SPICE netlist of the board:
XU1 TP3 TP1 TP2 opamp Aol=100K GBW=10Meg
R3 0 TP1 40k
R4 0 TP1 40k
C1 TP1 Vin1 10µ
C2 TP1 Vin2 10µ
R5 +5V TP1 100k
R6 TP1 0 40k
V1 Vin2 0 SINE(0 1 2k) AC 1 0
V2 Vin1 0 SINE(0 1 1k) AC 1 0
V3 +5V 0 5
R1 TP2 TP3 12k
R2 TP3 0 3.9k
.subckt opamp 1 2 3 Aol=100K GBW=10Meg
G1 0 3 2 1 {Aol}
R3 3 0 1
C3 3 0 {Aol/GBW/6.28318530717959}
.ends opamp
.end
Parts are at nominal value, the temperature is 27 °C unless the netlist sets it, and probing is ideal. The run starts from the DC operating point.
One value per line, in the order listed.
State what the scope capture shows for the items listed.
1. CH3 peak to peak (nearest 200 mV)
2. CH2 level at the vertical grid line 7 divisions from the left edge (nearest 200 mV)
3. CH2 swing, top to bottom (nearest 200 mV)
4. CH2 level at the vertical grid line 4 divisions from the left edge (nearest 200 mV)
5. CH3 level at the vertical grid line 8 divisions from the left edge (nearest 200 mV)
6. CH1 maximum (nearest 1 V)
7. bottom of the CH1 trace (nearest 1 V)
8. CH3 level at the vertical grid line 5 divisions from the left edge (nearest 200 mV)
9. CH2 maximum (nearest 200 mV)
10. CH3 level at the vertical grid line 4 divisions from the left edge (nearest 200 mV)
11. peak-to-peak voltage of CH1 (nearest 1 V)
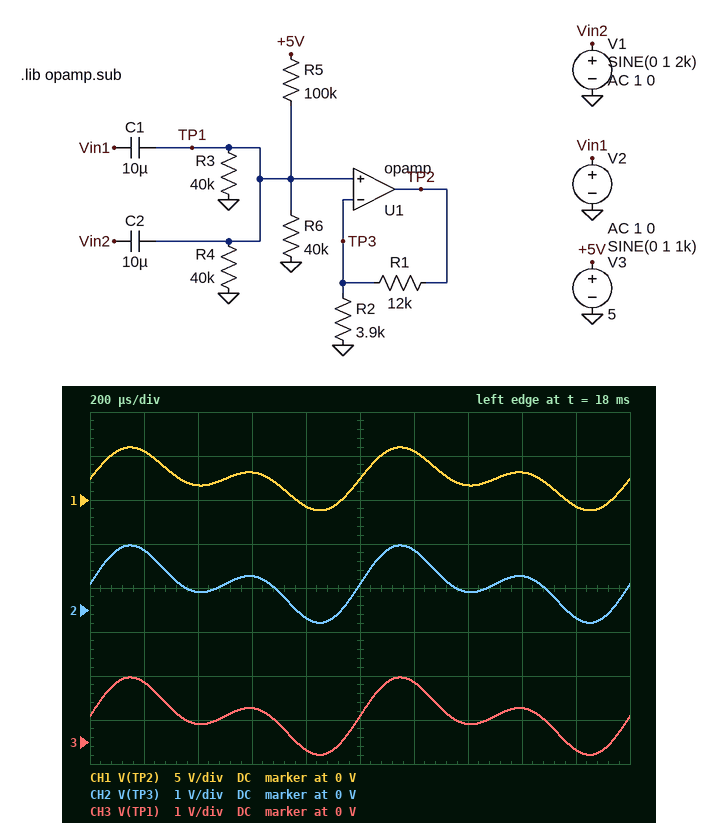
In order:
1.8 V
400 mV
1.8 V
-200 mV
800 mV
6 V
-1 V
600 mV
1.4 V
-200 mV
7 V
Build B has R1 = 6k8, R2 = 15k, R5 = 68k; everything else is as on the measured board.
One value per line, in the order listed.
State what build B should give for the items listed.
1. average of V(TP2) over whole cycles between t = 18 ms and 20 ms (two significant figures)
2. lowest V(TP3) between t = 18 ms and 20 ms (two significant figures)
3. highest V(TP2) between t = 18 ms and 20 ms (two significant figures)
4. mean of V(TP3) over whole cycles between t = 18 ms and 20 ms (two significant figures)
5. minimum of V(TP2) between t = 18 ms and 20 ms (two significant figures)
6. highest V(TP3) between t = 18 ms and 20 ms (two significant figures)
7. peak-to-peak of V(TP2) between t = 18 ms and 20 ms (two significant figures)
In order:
1.2 V
-61 mV
2.5 V
820 mV
-88 mV
1.7 V
2.6 V
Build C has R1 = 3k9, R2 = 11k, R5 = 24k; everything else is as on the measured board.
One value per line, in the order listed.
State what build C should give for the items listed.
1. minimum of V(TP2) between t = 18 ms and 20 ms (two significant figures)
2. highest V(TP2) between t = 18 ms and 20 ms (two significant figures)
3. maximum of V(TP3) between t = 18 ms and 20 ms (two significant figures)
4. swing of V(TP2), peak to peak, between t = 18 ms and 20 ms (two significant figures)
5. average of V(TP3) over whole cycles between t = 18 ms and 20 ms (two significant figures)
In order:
1.2 V
3.6 V
2.7 V
2.4 V
1.8 V
